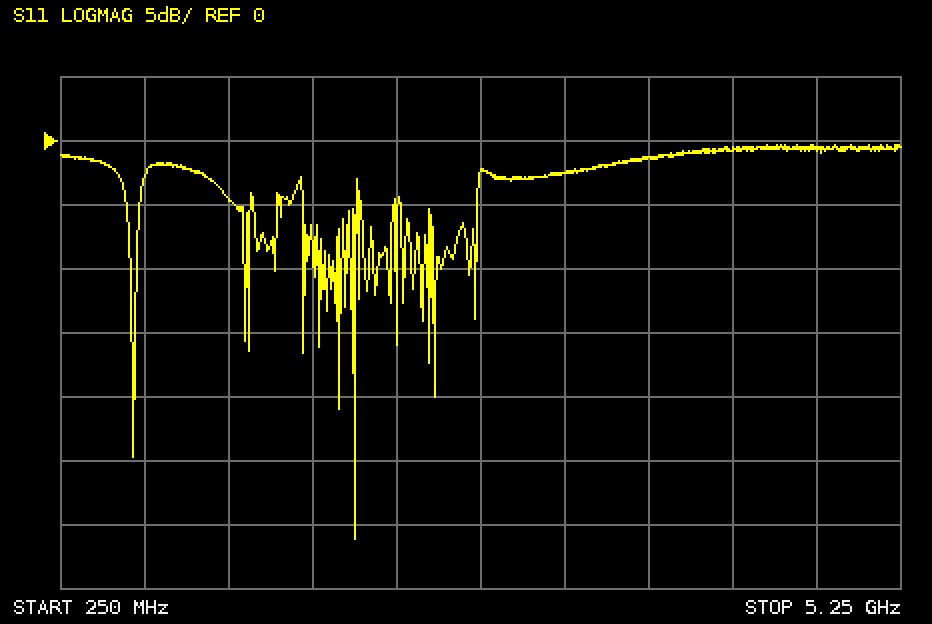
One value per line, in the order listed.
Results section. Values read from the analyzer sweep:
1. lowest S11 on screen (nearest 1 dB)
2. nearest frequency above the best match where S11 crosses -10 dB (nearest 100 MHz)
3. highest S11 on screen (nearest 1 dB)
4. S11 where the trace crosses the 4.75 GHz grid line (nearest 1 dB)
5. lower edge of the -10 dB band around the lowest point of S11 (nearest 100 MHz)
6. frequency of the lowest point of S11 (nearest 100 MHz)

-31 dB
2.0 GHz
0 dB
-1 dB
2.0 GHz
2.0 GHz
